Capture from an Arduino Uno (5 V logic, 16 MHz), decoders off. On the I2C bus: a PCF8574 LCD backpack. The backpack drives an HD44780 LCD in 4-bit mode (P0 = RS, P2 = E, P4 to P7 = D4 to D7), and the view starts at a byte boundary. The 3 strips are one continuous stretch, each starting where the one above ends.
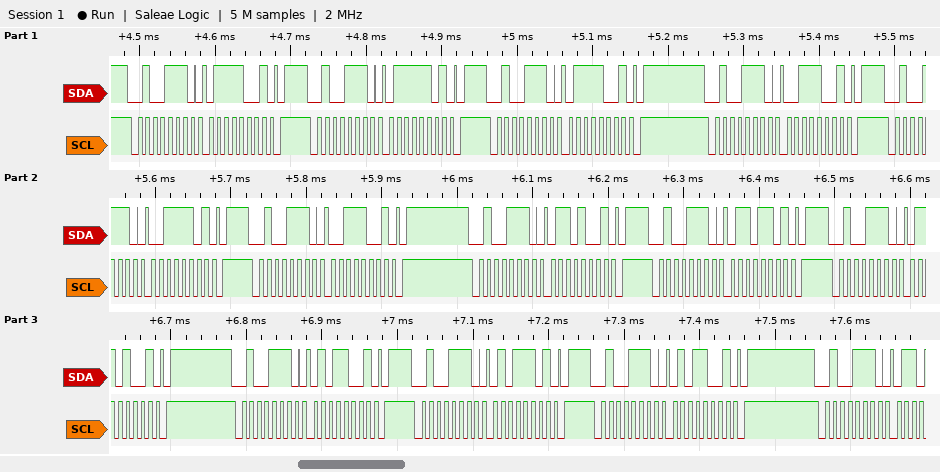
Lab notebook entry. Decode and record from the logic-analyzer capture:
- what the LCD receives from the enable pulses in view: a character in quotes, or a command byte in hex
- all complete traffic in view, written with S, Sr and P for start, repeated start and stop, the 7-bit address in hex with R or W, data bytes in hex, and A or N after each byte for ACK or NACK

's' 'e'
S 27W A 79 A P S 27W A 7D A P S 27W A 79 A P S 27W A 39 A P S 27W A 3D A P S 27W A 39 A P S 27W A 69 A P S 27W A 6D A P S 27W A 69 A P S 27W A 59 A P S 27W A 5D A P S 27W A 59 A P S 27W A
